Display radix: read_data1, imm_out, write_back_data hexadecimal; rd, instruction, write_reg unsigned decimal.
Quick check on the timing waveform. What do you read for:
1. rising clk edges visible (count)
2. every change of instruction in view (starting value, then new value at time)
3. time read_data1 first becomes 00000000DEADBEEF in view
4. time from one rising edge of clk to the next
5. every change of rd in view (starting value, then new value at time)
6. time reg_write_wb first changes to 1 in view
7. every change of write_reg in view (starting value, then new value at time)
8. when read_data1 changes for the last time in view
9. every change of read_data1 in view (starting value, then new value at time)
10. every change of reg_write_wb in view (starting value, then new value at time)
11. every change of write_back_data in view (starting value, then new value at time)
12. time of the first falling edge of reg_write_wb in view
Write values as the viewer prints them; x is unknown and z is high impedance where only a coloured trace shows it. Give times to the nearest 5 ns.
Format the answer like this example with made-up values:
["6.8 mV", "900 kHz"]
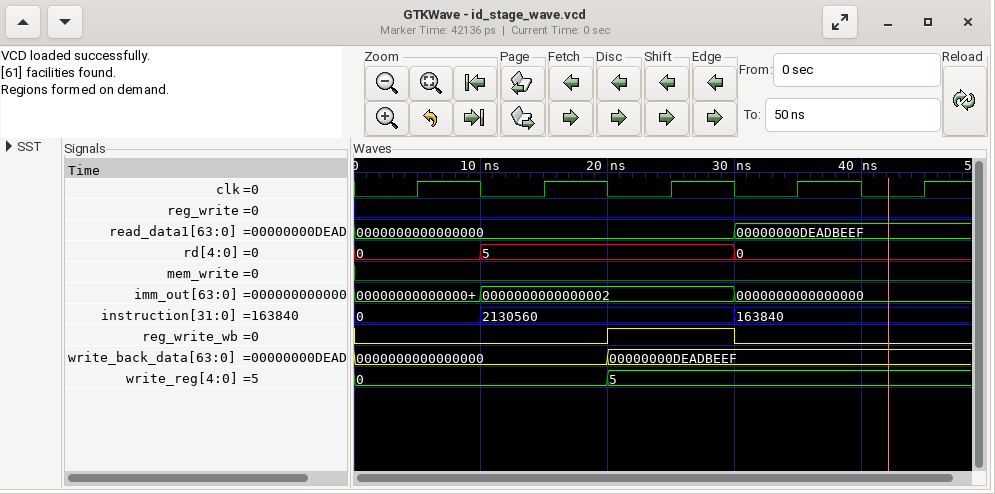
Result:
["5", "0, 2130560 at 10 ns, 163840 at 30 ns", "30 ns", "10 ns", "0, 5 at 10 ns, 0 at 30 ns", "20 ns", "0, 5 at 20 ns", "30 ns", "0000000000000000, 00000000DEADBEEF at 30 ns", "0, 1 at 20 ns, 0 at 30 ns", "0000000000000000, 00000000DEADBEEF at 20 ns", "30 ns"]
